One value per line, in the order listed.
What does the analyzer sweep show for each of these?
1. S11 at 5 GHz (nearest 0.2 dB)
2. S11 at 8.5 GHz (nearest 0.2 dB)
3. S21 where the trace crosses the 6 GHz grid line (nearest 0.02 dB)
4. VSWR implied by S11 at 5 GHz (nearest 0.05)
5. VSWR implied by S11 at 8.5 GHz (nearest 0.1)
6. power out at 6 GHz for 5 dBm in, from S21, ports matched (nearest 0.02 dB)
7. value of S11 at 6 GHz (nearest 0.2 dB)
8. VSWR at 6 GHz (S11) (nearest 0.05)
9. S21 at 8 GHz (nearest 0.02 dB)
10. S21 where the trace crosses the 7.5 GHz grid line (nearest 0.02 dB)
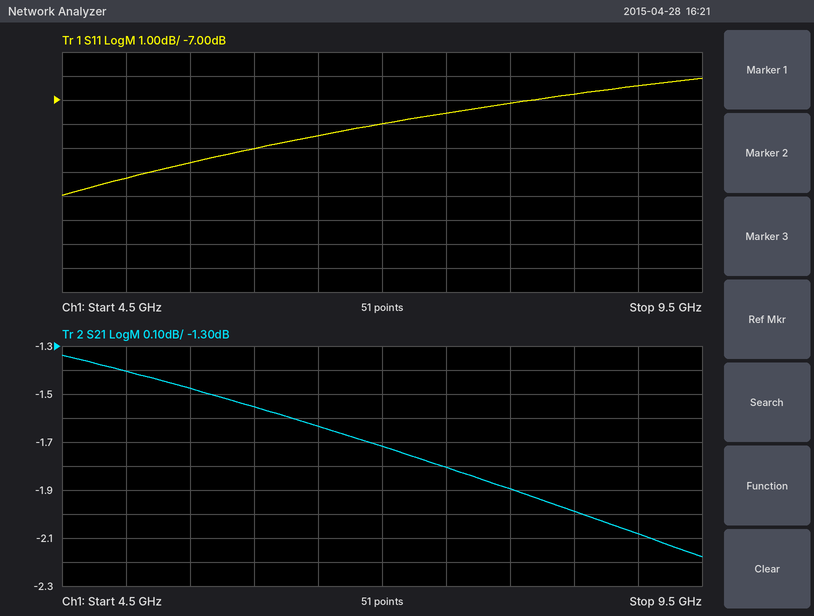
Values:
-10.2 dB
-6.8 dB
-1.56 dB
1.90
2.7
3.44 dBm
-9.0 dB
2.10
-1.90 dB
-1.80 dB
